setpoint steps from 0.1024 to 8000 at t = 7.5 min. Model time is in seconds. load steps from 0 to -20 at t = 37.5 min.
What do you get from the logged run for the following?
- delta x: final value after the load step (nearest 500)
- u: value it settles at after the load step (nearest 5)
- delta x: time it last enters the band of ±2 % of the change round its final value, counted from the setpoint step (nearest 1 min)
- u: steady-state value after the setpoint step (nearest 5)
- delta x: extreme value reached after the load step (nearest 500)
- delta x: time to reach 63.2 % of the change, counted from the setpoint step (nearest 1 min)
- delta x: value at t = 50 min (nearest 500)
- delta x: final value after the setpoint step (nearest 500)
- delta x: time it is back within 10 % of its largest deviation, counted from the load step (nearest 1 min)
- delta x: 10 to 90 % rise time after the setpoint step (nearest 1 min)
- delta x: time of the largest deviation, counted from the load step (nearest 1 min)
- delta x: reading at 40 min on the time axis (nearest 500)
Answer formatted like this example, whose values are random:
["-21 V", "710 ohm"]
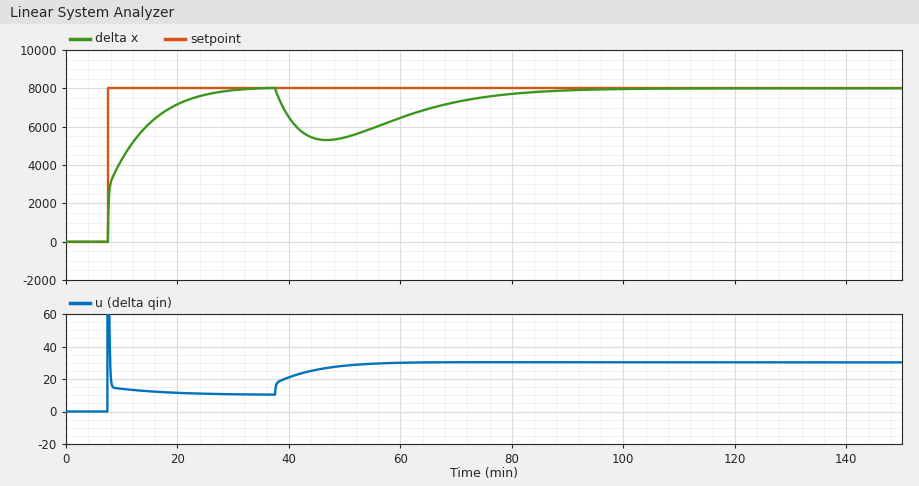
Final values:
["8000", "30", "21 min", "10", "5500", "4 min", "5500", "8000", "43 min", "13 min", "9 min", "6500"]
